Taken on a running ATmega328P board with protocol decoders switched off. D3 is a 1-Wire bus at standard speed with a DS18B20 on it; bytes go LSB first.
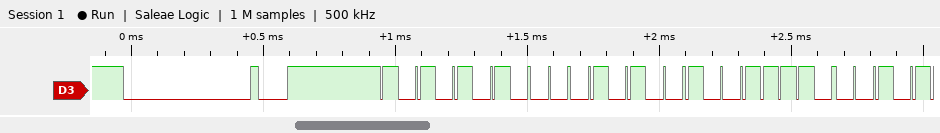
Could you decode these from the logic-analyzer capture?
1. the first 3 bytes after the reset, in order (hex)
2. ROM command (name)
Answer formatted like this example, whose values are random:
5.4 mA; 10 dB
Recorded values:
55 28 79; Match ROM
